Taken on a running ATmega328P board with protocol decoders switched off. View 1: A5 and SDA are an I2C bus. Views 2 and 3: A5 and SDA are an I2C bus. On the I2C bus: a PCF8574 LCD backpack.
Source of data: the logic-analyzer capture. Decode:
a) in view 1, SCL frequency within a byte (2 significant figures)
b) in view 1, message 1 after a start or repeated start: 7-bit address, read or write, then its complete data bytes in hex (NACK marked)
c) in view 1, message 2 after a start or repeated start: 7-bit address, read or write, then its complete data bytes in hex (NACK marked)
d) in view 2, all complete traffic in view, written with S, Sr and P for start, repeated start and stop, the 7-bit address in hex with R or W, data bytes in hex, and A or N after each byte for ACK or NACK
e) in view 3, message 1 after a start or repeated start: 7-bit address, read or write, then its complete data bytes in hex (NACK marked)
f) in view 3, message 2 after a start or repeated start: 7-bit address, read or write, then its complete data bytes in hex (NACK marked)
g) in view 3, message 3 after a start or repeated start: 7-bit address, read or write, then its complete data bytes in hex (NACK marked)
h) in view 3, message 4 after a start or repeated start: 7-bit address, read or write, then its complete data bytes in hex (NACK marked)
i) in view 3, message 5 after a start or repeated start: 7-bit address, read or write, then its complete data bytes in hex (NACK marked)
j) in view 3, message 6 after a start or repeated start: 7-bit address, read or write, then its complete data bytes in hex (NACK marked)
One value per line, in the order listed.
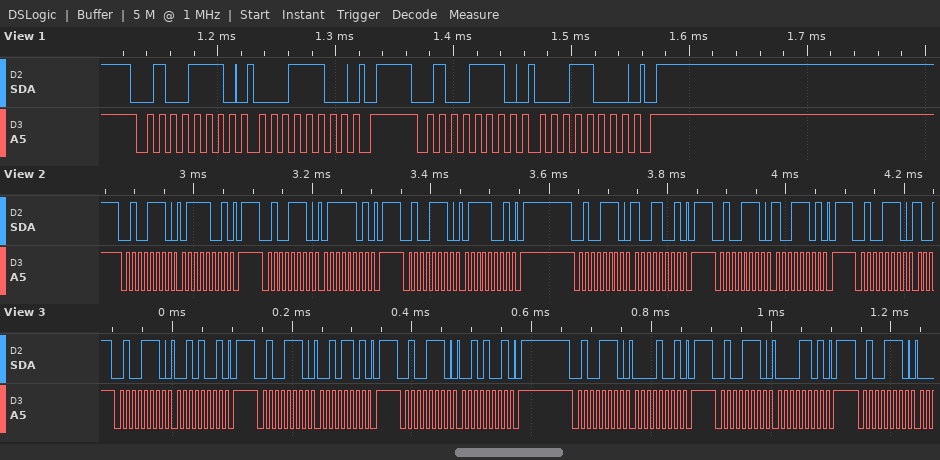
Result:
100 kHz
0x27 write: 1C
0x27 write: 18
S 27W A 79 A P S 27W A 7D A P S 27W A 79 A P S 27W A 99 A P S 27W A 9D A P S 27W A
0x27 write: 29
0x27 write: 2D
0x27 write: 29
0x27 write: 09
0x27 write: 0D
0x27 write
